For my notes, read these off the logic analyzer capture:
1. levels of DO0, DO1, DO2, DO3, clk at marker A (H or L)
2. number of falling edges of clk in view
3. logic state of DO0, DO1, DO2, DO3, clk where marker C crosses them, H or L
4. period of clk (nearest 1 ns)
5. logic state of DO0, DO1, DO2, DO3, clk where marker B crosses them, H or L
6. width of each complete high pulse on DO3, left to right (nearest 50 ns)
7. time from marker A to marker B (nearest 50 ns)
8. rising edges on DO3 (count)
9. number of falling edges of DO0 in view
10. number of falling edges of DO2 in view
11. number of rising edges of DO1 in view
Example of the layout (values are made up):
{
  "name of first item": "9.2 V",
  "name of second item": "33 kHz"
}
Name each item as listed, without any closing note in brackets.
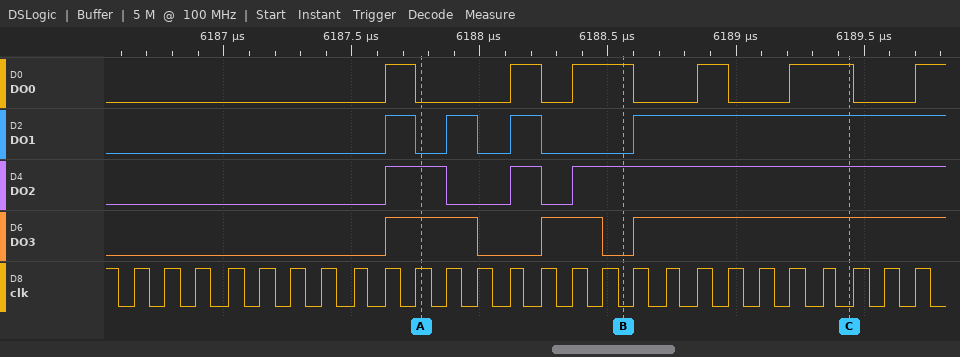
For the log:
{
  "levels of DO0, DO1, DO2, DO3, clk at marker A": "DO0=L, DO1=L, DO2=H, DO3=H, clk=H",
  "number of falling edges of clk in view": "27",
  "logic state of DO0, DO1, DO2, DO3, clk where marker C crosses them, H or L": "DO0=H, DO1=H, DO2=H, DO3=H, clk=L",
  "period of clk": "122 ns",
  "logic state of DO0, DO1, DO2, DO3, clk where marker B crosses them, H or L": "DO0=H, DO1=L, DO2=H, DO3=L, clk=L",
  "width of each complete high pulse on DO3, left to right": "350 ns, 250 ns",
  "time from marker A to marker B": "800 ns",
  "rising edges on DO3": "3",
  "number of falling edges of DO0 in view": "5",
  "number of falling edges of DO2 in view": "2",
  "number of rising edges of DO1 in view": "4"
}
